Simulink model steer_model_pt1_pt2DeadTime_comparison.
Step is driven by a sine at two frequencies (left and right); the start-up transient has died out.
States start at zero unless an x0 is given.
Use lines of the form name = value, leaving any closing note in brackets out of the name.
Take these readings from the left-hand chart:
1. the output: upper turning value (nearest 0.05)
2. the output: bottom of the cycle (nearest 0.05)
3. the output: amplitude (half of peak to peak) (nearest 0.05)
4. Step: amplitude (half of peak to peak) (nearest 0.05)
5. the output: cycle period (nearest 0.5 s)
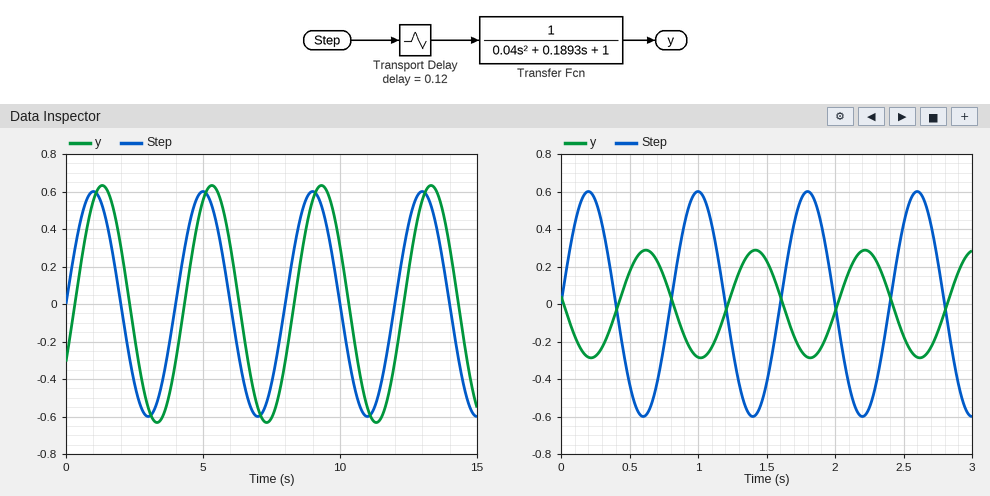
the output: upper turning value = 0.65
the output: bottom of the cycle = -0.65
the output: amplitude (half of peak to peak) = 0.65
Step: amplitude (half of peak to peak) = 0.60
the output: cycle period = 4.0 s
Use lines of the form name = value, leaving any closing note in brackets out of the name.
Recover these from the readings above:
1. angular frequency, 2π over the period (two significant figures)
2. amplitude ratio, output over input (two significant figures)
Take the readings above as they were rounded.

angular frequency, 2π over the period = 1.6 rad/s
amplitude ratio, output over input = 1.1
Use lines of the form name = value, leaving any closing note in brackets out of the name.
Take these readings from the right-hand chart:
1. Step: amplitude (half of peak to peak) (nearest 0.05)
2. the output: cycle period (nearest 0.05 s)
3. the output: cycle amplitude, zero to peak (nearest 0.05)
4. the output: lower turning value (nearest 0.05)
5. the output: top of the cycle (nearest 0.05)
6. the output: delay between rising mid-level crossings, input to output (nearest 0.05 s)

Step: amplitude (half of peak to peak) = 0.60
the output: cycle period = 0.80 s
the output: cycle amplitude, zero to peak = 0.30
the output: lower turning value = -0.30
the output: top of the cycle = 0.30
the output: delay between rising mid-level crossings, input to output = 0.40 s
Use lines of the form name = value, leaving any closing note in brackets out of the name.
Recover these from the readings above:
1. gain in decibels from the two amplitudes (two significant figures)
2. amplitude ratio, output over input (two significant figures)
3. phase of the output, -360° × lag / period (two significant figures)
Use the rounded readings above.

gain in decibels from the two amplitudes = -6.0 dB
amplitude ratio, output over input = 0.50
phase of the output, -360° × lag / period = -180°
